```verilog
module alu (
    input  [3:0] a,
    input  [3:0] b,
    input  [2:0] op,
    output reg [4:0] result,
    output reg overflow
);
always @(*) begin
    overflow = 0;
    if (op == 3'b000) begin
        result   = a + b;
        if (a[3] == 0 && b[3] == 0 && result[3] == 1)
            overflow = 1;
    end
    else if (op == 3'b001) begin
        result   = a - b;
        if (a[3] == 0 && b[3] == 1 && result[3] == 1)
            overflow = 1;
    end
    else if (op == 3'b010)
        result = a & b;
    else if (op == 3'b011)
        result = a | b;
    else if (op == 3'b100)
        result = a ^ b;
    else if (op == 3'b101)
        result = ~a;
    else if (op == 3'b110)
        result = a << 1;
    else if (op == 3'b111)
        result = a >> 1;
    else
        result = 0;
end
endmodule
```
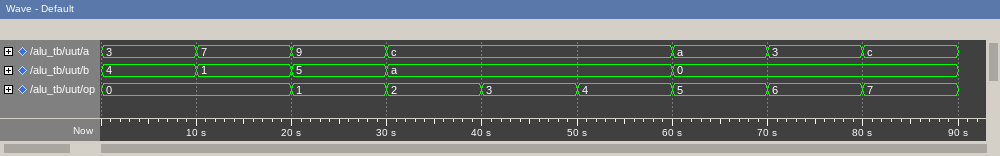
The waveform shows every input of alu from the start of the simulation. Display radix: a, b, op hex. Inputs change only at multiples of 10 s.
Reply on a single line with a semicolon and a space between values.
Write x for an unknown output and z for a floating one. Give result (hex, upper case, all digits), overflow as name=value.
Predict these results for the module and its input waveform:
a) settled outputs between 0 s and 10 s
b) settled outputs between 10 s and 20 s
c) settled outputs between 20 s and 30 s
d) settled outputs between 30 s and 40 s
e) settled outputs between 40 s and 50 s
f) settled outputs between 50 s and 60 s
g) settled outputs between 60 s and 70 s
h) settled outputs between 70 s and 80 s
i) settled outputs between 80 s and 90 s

result=07, overflow=0; result=08, overflow=1; result=04, overflow=0; result=08, overflow=0; result=0E, overflow=0; result=06, overflow=0; result=15, overflow=0; result=06, overflow=0; result=06, overflow=0
